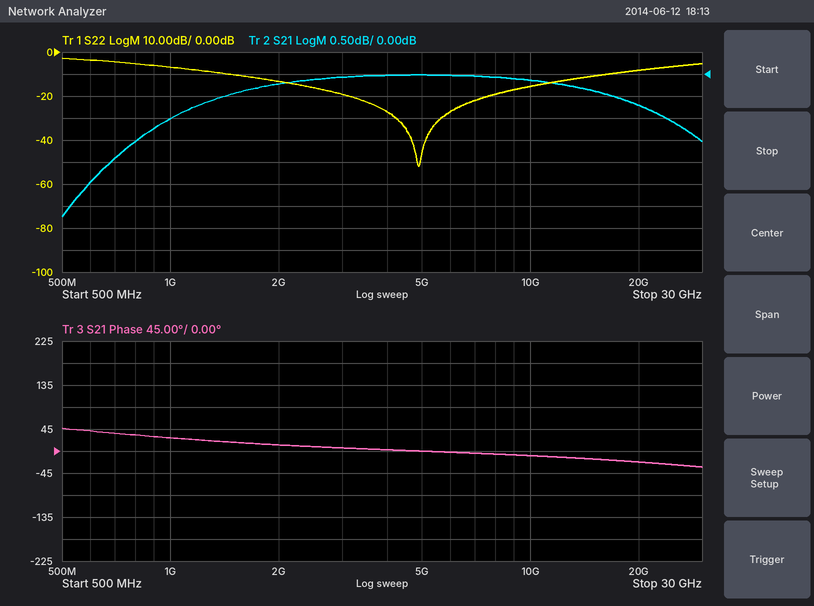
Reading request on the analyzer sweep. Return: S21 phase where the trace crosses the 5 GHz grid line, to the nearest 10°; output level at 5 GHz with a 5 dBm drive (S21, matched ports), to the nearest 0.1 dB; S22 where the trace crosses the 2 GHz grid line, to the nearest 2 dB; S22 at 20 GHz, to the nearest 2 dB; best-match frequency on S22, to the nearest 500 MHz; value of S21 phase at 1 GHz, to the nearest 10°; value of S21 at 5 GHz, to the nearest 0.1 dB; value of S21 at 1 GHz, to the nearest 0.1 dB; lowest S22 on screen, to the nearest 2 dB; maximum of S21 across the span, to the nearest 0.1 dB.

0°
5.0 dBm
-14 dB
-8 dB
5.0 GHz
30°
0.0 dB
-1.0 dB
-52 dB
0.0 dB
